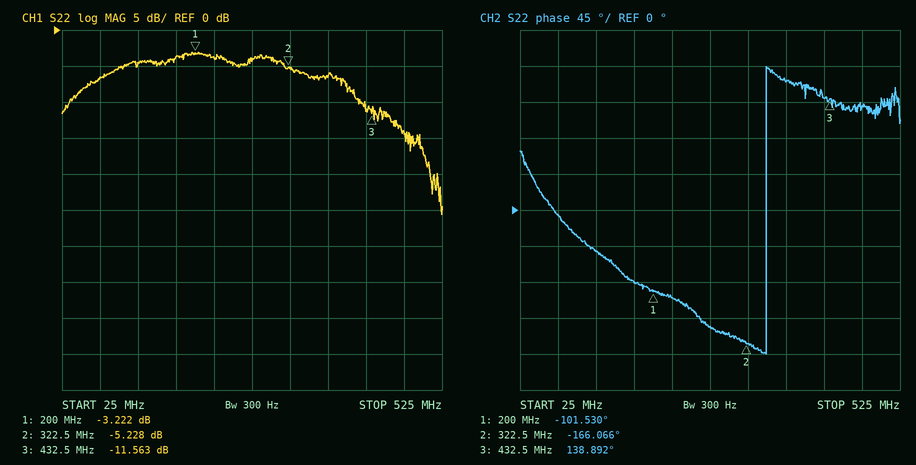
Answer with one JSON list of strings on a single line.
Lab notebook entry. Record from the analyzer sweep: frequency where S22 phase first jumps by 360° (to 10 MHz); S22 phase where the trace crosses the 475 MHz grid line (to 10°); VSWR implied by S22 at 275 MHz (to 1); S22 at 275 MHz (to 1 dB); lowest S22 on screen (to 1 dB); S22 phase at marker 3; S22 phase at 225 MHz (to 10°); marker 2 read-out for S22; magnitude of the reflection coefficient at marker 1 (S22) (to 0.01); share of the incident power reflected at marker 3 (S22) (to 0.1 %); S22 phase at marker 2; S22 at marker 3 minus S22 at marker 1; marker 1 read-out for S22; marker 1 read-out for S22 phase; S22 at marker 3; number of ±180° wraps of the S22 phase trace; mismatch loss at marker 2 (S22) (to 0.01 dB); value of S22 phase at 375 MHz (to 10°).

["350 MHz", "130°", "4", "-4 dB", "-26 dB", "138.892°", "-110°", "-5.228 dB", "0.69", "7.0 %", "-166.066°", "-8.341 dB", "-3.222 dB", "-101.530°", "-11.563 dB", "1", "1.55 dB", "160°"]
